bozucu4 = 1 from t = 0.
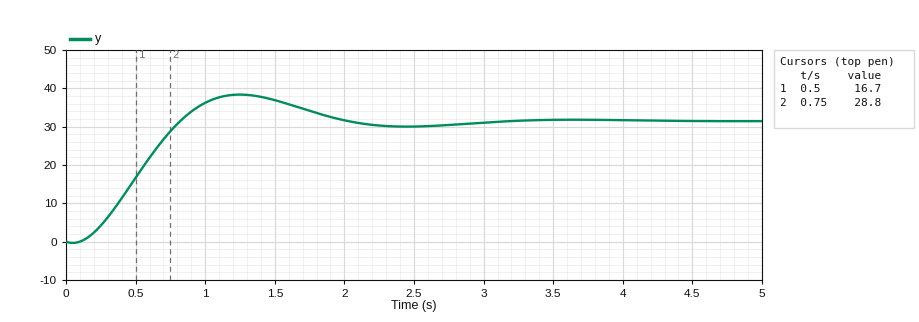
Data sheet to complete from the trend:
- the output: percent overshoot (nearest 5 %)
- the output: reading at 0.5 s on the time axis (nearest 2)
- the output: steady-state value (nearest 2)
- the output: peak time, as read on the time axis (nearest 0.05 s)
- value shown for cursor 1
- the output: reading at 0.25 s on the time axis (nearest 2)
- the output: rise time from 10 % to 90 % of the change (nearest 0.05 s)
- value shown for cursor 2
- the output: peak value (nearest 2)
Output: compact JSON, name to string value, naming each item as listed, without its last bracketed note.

{"the output: percent overshoot": "20 %", "the output: reading at 0.5 s on the time axis": "16", "the output: steady-state value": "32", "the output: peak time, as read on the time axis": "1.25 s", "value shown for cursor 1": "16.7", "the output: reading at 0.25 s on the time axis": "4", "the output: rise time from 10 % to 90 % of the change": "0.50 s", "value shown for cursor 2": "28.8", "the output: peak value": "38"}
